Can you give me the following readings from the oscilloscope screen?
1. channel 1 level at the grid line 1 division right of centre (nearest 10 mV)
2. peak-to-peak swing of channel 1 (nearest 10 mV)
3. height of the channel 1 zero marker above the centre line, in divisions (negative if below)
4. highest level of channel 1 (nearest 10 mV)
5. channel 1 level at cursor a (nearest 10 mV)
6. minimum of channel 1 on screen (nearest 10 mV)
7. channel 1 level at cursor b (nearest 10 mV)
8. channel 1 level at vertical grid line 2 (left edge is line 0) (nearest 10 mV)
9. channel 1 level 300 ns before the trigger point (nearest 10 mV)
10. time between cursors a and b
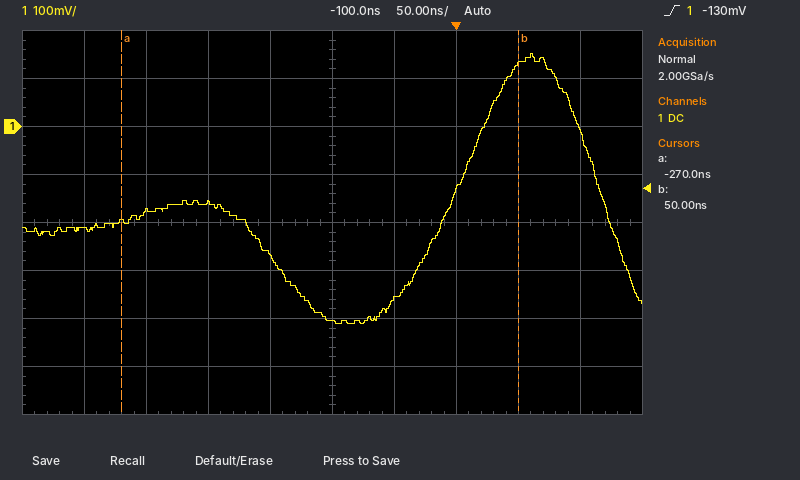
-360 mV
560 mV
+2.0 div
150 mV
-200 mV
-410 mV
130 mV
-180 mV
-210 mV
320 ns
